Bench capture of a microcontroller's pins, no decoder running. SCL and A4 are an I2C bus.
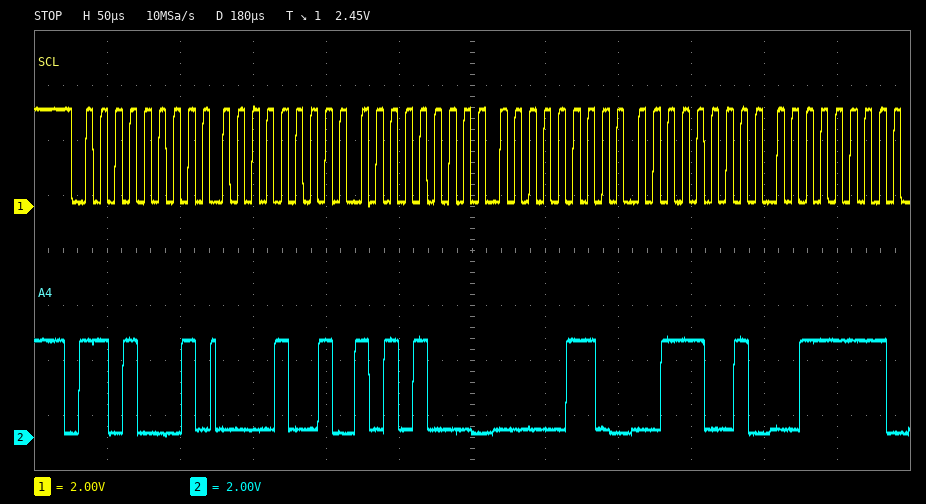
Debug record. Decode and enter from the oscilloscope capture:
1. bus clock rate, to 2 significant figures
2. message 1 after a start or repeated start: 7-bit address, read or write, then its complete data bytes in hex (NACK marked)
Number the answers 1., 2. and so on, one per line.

1. 100 kHz
2. 0x68 read: 09 A8 06 39 3F
